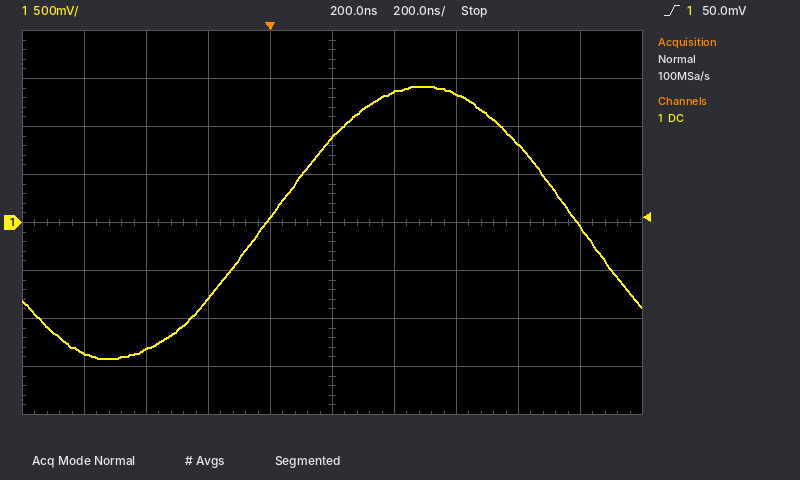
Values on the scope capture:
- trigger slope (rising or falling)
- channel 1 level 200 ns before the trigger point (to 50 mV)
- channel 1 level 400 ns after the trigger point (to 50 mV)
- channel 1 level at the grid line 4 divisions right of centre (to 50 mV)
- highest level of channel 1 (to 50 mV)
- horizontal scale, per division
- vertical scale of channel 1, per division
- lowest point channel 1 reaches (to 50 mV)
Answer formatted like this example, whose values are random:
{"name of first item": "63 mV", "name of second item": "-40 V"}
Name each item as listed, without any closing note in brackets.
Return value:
{"trigger slope": "rising", "channel 1 level 200 ns before the trigger point": "-800 mV", "channel 1 level 400 ns after the trigger point": "1.35 V", "channel 1 level at the grid line 4 divisions right of centre": "-50 mV", "highest level of channel 1": "1.40 V", "horizontal scale, per division": "200 ns", "vertical scale of channel 1, per division": "500 mV", "lowest point channel 1 reaches": "-1.40 V"}
